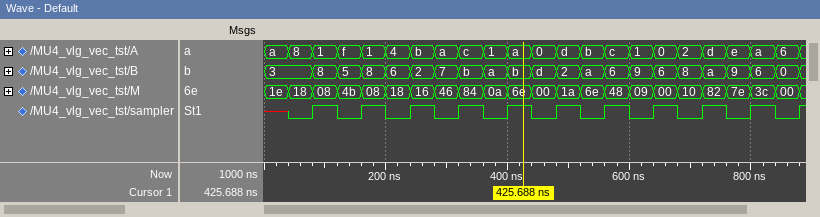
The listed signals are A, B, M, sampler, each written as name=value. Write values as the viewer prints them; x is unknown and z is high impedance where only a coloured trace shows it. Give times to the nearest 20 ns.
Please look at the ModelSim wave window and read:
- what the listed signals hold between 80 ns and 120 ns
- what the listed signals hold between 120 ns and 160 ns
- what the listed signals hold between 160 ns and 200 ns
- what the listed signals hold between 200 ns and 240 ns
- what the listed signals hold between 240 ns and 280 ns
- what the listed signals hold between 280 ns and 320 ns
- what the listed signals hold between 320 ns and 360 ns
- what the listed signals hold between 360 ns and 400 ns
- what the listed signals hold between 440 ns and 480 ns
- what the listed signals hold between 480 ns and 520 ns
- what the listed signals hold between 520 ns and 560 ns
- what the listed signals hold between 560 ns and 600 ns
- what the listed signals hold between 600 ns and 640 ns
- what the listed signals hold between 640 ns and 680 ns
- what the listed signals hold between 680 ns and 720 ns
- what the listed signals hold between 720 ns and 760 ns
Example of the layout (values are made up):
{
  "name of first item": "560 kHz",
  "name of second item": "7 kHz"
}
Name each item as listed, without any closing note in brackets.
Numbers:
{
  "what the listed signals hold between 80 ns and 120 ns": "A=1, B=8, M=08, sampler=1",
  "what the listed signals hold between 120 ns and 160 ns": "A=f, B=5, M=4b, sampler=0",
  "what the listed signals hold between 160 ns and 200 ns": "A=1, B=8, M=08, sampler=1",
  "what the listed signals hold between 200 ns and 240 ns": "A=4, B=6, M=18, sampler=0",
  "what the listed signals hold between 240 ns and 280 ns": "A=b, B=2, M=16, sampler=1",
  "what the listed signals hold between 280 ns and 320 ns": "A=a, B=7, M=46, sampler=0",
  "what the listed signals hold between 320 ns and 360 ns": "A=c, B=b, M=84, sampler=1",
  "what the listed signals hold between 360 ns and 400 ns": "A=1, B=a, M=0a, sampler=0",
  "what the listed signals hold between 440 ns and 480 ns": "A=0, B=d, M=00, sampler=0",
  "what the listed signals hold between 480 ns and 520 ns": "A=d, B=2, M=1a, sampler=1",
  "what the listed signals hold between 520 ns and 560 ns": "A=b, B=a, M=6e, sampler=0",
  "what the listed signals hold between 560 ns and 600 ns": "A=c, B=6, M=48, sampler=1",
  "what the listed signals hold between 600 ns and 640 ns": "A=1, B=9, M=09, sampler=0",
  "what the listed signals hold between 640 ns and 680 ns": "A=0, B=6, M=00, sampler=1",
  "what the listed signals hold between 680 ns and 720 ns": "A=2, B=8, M=10, sampler=0",
  "what the listed signals hold between 720 ns and 760 ns": "A=d, B=a, M=82, sampler=1"
}
